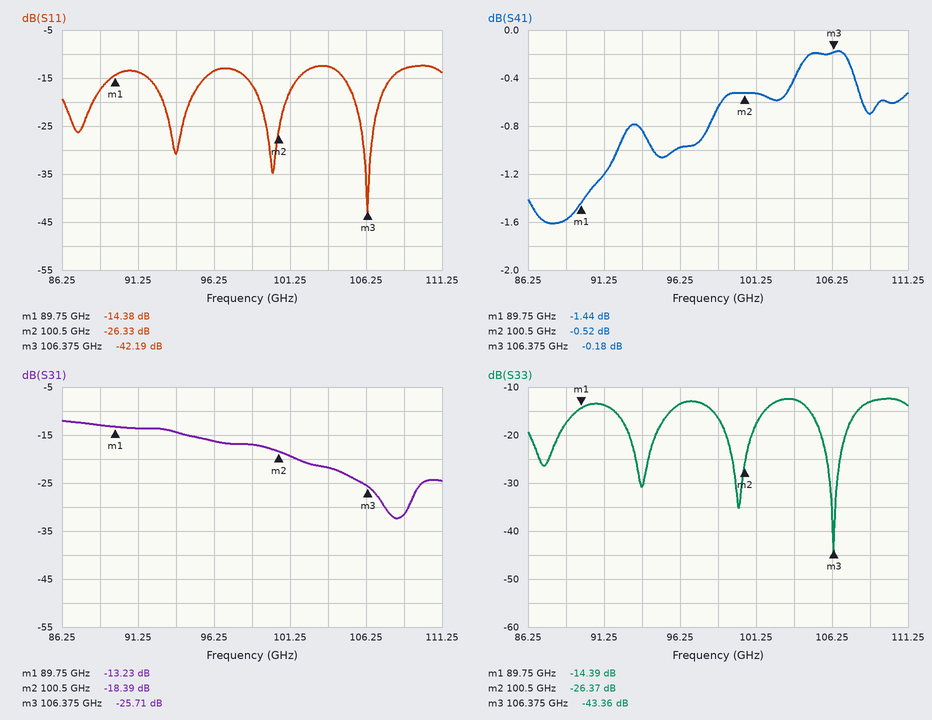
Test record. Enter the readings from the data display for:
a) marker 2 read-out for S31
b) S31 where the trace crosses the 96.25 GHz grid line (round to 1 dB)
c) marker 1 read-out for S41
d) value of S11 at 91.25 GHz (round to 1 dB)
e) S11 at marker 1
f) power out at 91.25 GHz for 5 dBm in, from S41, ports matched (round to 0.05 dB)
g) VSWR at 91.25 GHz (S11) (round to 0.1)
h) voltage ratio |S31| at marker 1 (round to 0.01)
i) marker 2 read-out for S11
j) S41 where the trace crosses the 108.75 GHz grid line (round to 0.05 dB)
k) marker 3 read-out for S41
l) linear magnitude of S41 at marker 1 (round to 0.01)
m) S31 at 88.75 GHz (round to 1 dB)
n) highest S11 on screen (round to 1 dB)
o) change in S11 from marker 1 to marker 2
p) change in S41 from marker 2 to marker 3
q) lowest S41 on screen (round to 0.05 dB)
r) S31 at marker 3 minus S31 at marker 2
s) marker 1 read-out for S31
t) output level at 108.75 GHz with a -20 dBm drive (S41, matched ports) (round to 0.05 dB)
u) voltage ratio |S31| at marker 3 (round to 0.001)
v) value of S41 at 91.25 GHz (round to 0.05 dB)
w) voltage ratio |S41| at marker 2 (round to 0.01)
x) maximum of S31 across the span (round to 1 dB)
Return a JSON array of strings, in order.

["-18.39 dB", "-16 dB", "-1.44 dB", "-14 dB", "-14.38 dB", "3.80 dBm", "1.5", "0.22", "-26.33 dB", "-0.70 dB", "-0.18 dB", "0.85", "-13 dB", "-12 dB", "-11.95 dB", "0.34 dB", "-1.60 dB", "-7.32 dB", "-13.23 dB", "-20.70 dBm", "0.052", "-1.20 dB", "0.94", "-12 dB"]
